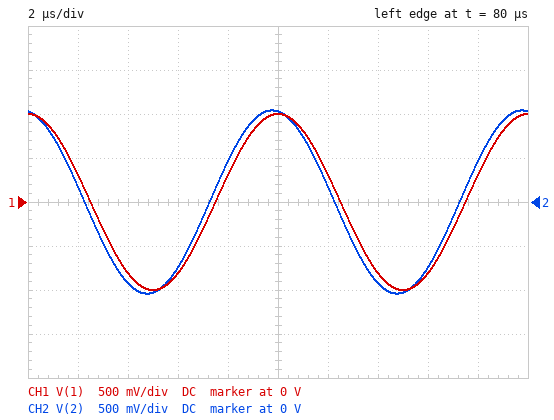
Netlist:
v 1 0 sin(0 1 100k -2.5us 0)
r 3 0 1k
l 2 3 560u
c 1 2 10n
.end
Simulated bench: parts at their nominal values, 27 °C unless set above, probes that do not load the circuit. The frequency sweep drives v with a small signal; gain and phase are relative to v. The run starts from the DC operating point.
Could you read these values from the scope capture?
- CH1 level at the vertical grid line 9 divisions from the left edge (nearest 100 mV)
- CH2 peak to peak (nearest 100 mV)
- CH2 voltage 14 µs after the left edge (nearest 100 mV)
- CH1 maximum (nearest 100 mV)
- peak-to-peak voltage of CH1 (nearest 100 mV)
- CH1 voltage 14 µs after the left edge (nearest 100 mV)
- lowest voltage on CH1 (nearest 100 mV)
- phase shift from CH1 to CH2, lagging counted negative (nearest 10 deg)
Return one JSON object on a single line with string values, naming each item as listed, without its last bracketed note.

{"CH1 level at the vertical grid line 9 divisions from the left edge": "300 mV", "CH2 peak to peak": "2.1 V", "CH2 voltage 14 µs after the left edge": "-900 mV", "CH1 maximum": "1.0 V", "peak-to-peak voltage of CH1": "2.0 V", "CH1 voltage 14 µs after the left edge": "-800 mV", "lowest voltage on CH1": "-1.0 V", "phase shift from CH1 to CH2, lagging counted negative": "10 deg"}
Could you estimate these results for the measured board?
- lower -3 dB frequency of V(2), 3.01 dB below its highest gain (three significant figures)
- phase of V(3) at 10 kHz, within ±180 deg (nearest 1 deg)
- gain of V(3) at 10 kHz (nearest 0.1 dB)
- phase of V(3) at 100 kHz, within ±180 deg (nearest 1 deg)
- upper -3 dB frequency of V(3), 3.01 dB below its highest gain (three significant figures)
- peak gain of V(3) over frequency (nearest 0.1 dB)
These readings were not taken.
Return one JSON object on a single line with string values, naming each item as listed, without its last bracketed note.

{"lower -3 dB frequency of V(2), 3.01 dB below its highest gain": "16.3 kHz", "phase of V(3) at 10 kHz, within ±180 deg": "57 deg", "gain of V(3) at 10 kHz": "-5.3 dB", "phase of V(3) at 100 kHz, within ±180 deg": "-11 deg", "upper -3 dB frequency of V(3), 3.01 dB below its highest gain": "299 kHz", "peak gain of V(3) over frequency": "0 dB"}
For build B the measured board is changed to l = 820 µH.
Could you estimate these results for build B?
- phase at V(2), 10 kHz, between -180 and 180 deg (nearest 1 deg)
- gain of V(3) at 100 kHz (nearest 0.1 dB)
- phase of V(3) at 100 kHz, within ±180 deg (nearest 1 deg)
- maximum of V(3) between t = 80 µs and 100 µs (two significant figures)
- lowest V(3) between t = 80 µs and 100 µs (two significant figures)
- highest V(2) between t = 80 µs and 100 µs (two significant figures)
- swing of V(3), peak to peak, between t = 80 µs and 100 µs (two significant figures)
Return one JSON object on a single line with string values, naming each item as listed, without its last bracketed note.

{"phase at V(2), 10 kHz, between -180 and 180 deg": "60 deg", "gain of V(3) at 100 kHz": "-0.5 dB", "phase of V(3) at 100 kHz, within ±180 deg": "-20 deg", "maximum of V(3) between t = 80 µs and 100 µs": "940 mV", "lowest V(3) between t = 80 µs and 100 µs": "-940 mV", "highest V(2) between t = 80 µs and 100 µs": "1.1 V", "swing of V(3), peak to peak, between t = 80 µs and 100 µs": "1.9 V"}
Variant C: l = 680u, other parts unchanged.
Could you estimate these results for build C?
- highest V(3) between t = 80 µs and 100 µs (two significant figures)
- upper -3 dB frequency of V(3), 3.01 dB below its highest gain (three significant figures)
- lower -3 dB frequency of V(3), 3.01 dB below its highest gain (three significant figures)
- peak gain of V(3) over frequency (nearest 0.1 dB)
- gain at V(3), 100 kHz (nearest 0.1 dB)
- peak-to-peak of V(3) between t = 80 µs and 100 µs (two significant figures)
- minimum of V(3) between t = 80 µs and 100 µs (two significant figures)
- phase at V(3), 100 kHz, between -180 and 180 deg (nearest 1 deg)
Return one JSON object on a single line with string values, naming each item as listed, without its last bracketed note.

{"highest V(3) between t = 80 µs and 100 µs": "970 mV", "upper -3 dB frequency of V(3), 3.01 dB below its highest gain": "249 kHz", "lower -3 dB frequency of V(3), 3.01 dB below its highest gain": "15.0 kHz", "peak gain of V(3) over frequency": "0 dB", "gain at V(3), 100 kHz": "-0.3 dB", "peak-to-peak of V(3) between t = 80 µs and 100 µs": "1.9 V", "minimum of V(3) between t = 80 µs and 100 µs": "-970 mV", "phase at V(3), 100 kHz, between -180 and 180 deg": "-15 deg"}
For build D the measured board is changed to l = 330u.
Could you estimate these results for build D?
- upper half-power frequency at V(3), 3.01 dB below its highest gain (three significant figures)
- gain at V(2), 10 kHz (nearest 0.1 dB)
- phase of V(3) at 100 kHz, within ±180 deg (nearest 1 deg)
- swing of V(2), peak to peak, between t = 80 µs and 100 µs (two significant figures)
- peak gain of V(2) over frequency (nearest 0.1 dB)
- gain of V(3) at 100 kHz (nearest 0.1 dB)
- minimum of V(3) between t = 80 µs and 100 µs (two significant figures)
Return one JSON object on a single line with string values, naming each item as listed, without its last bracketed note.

{"upper half-power frequency at V(3), 3.01 dB below its highest gain": "498 kHz", "gain at V(2), 10 kHz": "-5.4 dB", "phase of V(3) at 100 kHz, within ±180 deg": "-3 deg", "swing of V(2), peak to peak, between t = 80 µs and 100 µs": "2.0 V", "peak gain of V(2) over frequency": "0.2 dB", "gain of V(3) at 100 kHz": "0 dB", "minimum of V(3) between t = 80 µs and 100 µs": "-1.0 V"}
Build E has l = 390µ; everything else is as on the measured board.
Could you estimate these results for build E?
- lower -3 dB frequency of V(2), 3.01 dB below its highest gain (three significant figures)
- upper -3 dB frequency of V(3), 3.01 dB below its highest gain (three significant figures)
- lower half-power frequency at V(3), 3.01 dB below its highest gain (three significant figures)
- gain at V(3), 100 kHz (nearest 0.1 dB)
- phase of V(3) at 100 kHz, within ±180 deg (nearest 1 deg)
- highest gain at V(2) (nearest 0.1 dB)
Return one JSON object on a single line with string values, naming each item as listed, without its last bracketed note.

{"lower -3 dB frequency of V(2), 3.01 dB below its highest gain": "16.2 kHz", "upper -3 dB frequency of V(3), 3.01 dB below its highest gain": "423 kHz", "lower half-power frequency at V(3), 3.01 dB below its highest gain": "15.3 kHz", "gain at V(3), 100 kHz": "0 dB", "phase of V(3) at 100 kHz, within ±180 deg": "-5 deg", "highest gain at V(2)": "0.3 dB"}
